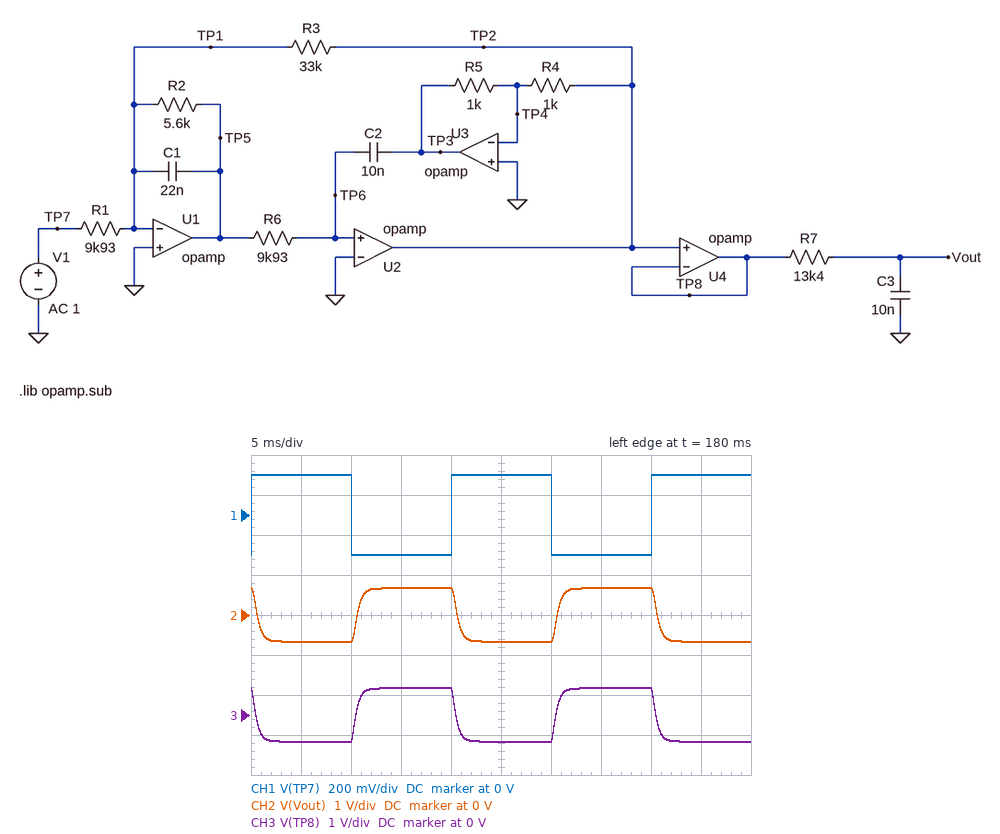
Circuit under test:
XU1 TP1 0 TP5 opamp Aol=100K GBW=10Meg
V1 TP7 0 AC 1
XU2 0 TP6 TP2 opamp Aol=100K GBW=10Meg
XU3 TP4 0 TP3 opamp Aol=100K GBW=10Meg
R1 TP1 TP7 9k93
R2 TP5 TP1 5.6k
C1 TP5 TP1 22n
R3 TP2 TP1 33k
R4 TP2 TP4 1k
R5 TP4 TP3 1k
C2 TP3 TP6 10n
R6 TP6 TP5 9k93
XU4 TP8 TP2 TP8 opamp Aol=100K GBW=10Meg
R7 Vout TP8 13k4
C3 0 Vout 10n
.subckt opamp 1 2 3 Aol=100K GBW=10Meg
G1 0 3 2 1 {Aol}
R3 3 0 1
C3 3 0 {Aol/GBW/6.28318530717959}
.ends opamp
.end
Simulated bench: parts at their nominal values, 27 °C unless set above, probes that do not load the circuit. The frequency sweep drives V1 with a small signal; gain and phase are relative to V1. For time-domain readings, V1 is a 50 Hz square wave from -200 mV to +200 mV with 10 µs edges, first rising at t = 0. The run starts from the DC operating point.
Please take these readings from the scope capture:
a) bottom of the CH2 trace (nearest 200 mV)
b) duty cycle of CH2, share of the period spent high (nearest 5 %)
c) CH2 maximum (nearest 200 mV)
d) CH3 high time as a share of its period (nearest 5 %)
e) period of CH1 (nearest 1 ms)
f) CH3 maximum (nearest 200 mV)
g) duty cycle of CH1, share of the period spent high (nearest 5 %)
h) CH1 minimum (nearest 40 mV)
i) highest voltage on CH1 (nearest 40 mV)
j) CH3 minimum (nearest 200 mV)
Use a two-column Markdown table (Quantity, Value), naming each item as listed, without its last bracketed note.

| Quantity | Value |
|---|---|
| bottom of the CH2 trace | -600 mV |
| duty cycle of CH2, share of the period spent high | 50 % |
| CH2 maximum | 600 mV |
| CH3 high time as a share of its period | 50 % |
| period of CH1 | 20 ms |
| CH3 maximum | 600 mV |
| duty cycle of CH1, share of the period spent high | 50 % |
| CH1 minimum | -200 mV |
| highest voltage on CH1 | 200 mV |
| CH3 minimum | -600 mV |
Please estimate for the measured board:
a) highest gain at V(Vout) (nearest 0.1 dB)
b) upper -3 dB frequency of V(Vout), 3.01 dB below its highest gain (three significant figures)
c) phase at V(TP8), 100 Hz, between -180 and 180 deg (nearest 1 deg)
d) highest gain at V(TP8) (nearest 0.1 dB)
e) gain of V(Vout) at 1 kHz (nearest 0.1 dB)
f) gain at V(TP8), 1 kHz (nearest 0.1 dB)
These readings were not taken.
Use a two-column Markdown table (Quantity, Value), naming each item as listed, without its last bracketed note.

| Quantity | Value |
|---|---|
| highest gain at V(Vout) | 10.4 dB |
| upper -3 dB frequency of V(Vout), 3.01 dB below its highest gain | 317 Hz |
| phase at V(TP8), 100 Hz, between -180 and 180 deg | 159 deg |
| highest gain at V(TP8) | 10.4 dB |
| gain of V(Vout) at 1 kHz | -4.2 dB |
| gain at V(TP8), 1 kHz | -1.9 dB |
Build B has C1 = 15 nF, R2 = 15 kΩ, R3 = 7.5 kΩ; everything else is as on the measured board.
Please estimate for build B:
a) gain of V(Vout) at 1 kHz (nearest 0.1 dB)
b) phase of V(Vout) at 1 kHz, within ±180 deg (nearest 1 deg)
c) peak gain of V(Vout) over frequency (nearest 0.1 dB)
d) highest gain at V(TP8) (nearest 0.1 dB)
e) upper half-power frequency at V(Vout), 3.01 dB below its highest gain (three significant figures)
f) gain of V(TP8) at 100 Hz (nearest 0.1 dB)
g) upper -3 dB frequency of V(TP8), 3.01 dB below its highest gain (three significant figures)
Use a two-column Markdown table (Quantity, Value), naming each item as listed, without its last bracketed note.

| Quantity | Value |
|---|---|
| gain of V(Vout) at 1 kHz | -0.9 dB |
| phase of V(Vout) at 1 kHz, within ±180 deg | 111 deg |
| peak gain of V(Vout) over frequency | 0.6 dB |
| highest gain at V(TP8) | 4.4 dB |
| upper half-power frequency at V(Vout), 3.01 dB below its highest gain | 1.68 kHz |
| gain of V(TP8) at 100 Hz | -2.4 dB |
| upper -3 dB frequency of V(TP8), 3.01 dB below its highest gain | 1.75 kHz |
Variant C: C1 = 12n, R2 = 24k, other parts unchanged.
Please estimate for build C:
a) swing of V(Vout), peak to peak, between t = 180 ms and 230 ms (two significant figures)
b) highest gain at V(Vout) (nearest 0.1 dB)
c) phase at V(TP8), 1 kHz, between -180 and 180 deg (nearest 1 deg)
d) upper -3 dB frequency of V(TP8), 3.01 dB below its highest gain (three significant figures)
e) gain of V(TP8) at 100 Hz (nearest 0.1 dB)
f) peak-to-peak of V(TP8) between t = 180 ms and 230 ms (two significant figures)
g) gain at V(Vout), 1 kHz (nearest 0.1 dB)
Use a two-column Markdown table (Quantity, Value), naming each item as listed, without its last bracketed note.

| Quantity | Value |
|---|---|
| swing of V(Vout), peak to peak, between t = 180 ms and 230 ms | 2.0 V |
| highest gain at V(Vout) | 13.0 dB |
| phase at V(TP8), 1 kHz, between -180 and 180 deg | 57 deg |
| upper -3 dB frequency of V(TP8), 3.01 dB below its highest gain | 953 Hz |
| gain of V(TP8) at 100 Hz | 10.5 dB |
| peak-to-peak of V(TP8) between t = 180 ms and 230 ms | 2.2 V |
| gain at V(Vout), 1 kHz | 7.9 dB |
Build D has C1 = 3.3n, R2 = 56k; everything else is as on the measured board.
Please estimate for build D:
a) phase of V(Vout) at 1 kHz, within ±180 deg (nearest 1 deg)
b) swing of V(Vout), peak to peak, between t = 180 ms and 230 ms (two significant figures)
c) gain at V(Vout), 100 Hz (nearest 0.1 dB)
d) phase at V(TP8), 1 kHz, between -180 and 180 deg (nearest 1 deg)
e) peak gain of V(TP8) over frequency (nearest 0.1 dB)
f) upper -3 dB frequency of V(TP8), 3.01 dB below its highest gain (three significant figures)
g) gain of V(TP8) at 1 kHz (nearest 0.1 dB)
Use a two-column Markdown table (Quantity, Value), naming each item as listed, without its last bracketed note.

| Quantity | Value |
|---|---|
| phase of V(Vout) at 1 kHz, within ±180 deg | 107 deg |
| swing of V(Vout), peak to peak, between t = 180 ms and 230 ms | 1.8 V |
| gain at V(Vout), 100 Hz | 10.4 dB |
| phase at V(TP8), 1 kHz, between -180 and 180 deg | 147 deg |
| peak gain of V(TP8) over frequency | 15.8 dB |
| upper -3 dB frequency of V(TP8), 3.01 dB below its highest gain | 1.80 kHz |
| gain of V(TP8) at 1 kHz | 13.8 dB |
